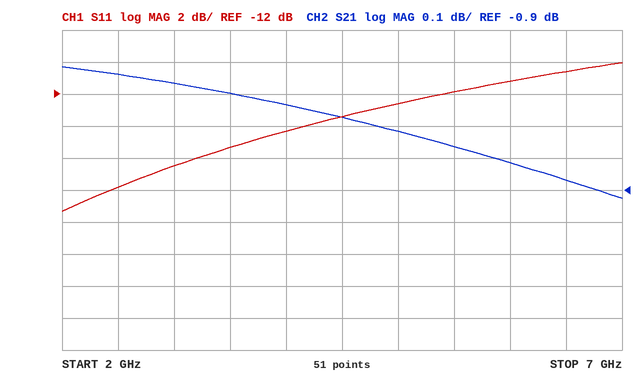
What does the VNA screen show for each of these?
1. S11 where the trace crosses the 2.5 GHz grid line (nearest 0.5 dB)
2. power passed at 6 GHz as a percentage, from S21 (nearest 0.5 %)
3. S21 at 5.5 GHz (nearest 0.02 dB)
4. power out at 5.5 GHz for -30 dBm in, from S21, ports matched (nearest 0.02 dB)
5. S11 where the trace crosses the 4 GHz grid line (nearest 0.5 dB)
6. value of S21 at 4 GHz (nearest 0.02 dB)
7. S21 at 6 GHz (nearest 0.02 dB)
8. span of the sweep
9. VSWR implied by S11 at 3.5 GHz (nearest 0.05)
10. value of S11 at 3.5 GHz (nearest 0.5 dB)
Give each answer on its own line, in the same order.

-18.0 dB
83.0 %
-0.76 dB
-30.76 dBm
-14.5 dB
-0.64 dB
-0.82 dB
5 GHz
1.40
-15.5 dB
